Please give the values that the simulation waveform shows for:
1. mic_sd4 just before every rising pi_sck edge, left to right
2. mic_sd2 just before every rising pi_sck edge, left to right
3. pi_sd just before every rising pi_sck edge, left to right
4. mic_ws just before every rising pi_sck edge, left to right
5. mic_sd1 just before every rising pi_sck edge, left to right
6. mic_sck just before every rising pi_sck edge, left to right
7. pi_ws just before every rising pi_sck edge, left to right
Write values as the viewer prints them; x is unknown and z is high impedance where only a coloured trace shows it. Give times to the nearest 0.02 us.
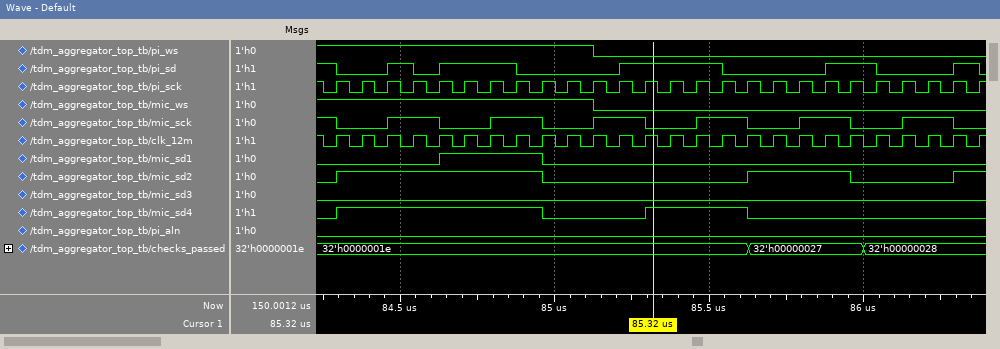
0 1 1 1 1 1 1 1 1 0 0 0 0 1 1 1 1 0 0 0 0 0 0 0 0 0
0 1 1 1 1 1 1 1 1 0 0 0 0 0 0 0 0 1 1 1 1 0 0 0 0 1
1 0 0 1 0 1 1 1 0 0 0 0 1 1 1 1 0 0 0 0 1 1 0 0 0 1
1 1 1 1 1 1 1 1 1 1 1 0 0 0 0 0 0 0 0 0 0 0 0 0 0 0
0 0 0 0 0 1 1 1 1 0 0 0 0 0 0 0 0 0 0 0 0 0 0 0 0 0
1 0 0 1 1 0 0 1 1 0 0 1 1 0 0 1 1 0 0 1 1 0 0 1 1 0
1 1 1 1 1 1 1 1 1 1 1 0 0 0 0 0 0 0 0 0 0 0 0 0 0 0
